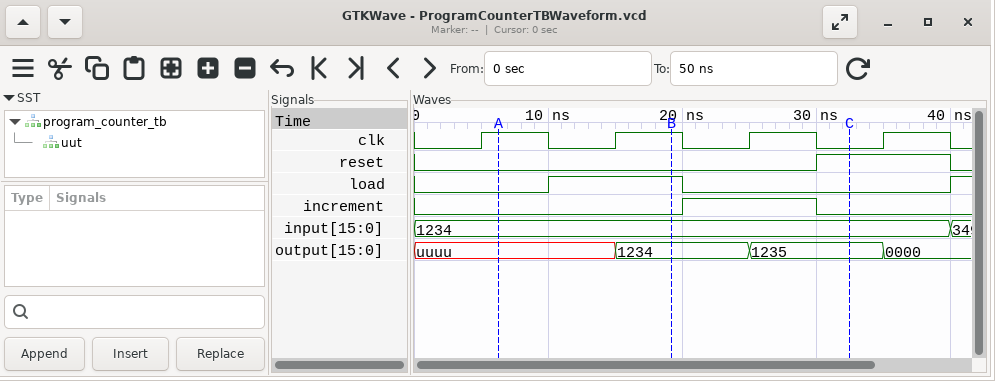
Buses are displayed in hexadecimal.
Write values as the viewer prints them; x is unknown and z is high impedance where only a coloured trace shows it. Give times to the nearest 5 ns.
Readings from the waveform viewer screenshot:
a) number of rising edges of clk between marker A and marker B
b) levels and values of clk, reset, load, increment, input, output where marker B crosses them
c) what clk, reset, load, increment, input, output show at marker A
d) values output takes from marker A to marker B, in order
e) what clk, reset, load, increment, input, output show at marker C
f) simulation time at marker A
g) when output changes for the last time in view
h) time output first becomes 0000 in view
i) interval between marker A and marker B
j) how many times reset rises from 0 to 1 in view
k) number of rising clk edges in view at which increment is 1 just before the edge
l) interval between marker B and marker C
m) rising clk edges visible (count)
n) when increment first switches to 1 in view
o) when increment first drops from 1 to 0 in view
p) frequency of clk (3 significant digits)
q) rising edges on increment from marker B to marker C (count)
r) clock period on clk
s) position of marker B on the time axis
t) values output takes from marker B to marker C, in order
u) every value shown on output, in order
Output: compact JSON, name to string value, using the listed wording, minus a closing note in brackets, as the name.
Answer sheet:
{"number of rising edges of clk between marker A and marker B": "1", "levels and values of clk, reset, load, increment, input, output where marker B crosses them": "clk=1, reset=0, load=1, increment=0, input=1234, output=1234", "what clk, reset, load, increment, input, output show at marker A": "clk=1, reset=0, load=0, increment=0, input=1234, output=uuuu", "values output takes from marker A to marker B, in order": "uuuu, 1234", "what clk, reset, load, increment, input, output show at marker C": "clk=0, reset=1, load=0, increment=0, input=1234, output=1235", "simulation time at marker A": "5 ns", "when output changes for the last time in view": "35 ns", "time output first becomes 0000 in view": "35 ns", "interval between marker A and marker B": "15 ns", "how many times reset rises from 0 to 1 in view": "1", "number of rising clk edges in view at which increment is 1 just before the edge": "1", "interval between marker B and marker C": "15 ns", "rising clk edges visible": "4", "when increment first switches to 1 in view": "20 ns", "when increment first drops from 1 to 0 in view": "30 ns", "frequency of clk": "100 MHz", "rising edges on increment from marker B to marker C": "1", "clock period on clk": "10 ns", "position of marker B on the time axis": "20 ns", "values output takes from marker B to marker C, in order": "1234, 1235", "every value shown on output, in order": "uuuu, 1234, 1235, 0000"}
